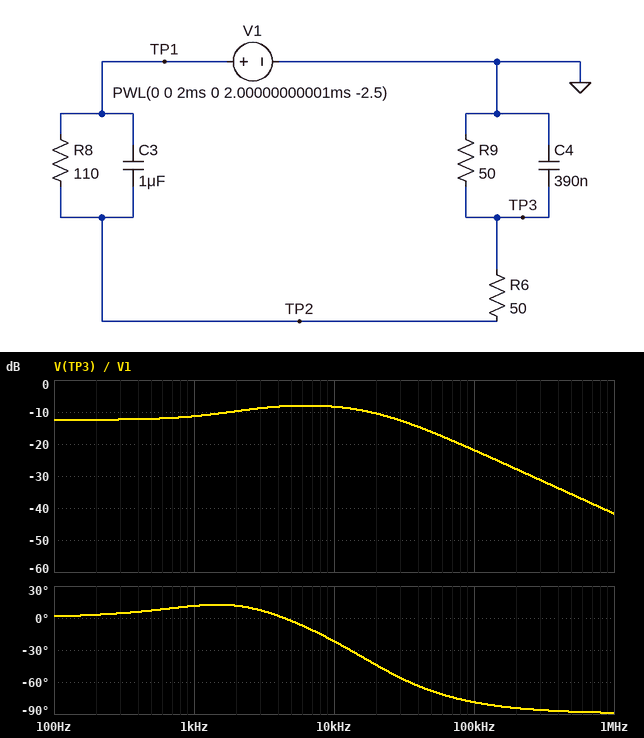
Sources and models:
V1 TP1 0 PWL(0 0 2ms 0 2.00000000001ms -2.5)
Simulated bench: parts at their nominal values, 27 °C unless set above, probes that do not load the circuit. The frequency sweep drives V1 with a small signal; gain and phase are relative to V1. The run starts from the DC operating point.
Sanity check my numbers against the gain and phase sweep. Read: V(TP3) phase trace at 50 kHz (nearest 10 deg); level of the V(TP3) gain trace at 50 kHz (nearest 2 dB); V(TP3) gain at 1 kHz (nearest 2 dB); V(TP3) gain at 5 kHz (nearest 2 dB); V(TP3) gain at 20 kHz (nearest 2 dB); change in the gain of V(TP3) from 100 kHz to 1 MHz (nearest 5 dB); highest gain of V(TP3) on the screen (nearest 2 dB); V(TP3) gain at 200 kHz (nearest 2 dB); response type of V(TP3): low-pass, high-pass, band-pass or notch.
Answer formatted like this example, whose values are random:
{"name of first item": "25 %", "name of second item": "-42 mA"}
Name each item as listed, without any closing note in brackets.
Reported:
{"V(TP3) phase trace at 50 kHz": "-70 deg", "level of the V(TP3) gain trace at 50 kHz": "-16 dB", "V(TP3) gain at 1 kHz": "-12 dB", "V(TP3) gain at 5 kHz": "-8 dB", "V(TP3) gain at 20 kHz": "-10 dB", "change in the gain of V(TP3) from 100 kHz to 1 MHz": "-20 dB", "highest gain of V(TP3) on the screen": "-8 dB", "V(TP3) gain at 200 kHz": "-28 dB", "response type of V(TP3): low-pass, high-pass, band-pass or notch": "low-pass"}
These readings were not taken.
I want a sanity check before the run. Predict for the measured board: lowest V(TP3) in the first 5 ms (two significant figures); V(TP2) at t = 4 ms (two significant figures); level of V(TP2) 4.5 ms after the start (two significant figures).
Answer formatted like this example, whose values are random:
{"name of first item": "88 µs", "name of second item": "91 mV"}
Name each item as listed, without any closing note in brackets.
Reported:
{"lowest V(TP3) in the first 5 ms": "-930 mV", "V(TP2) at t = 4 ms": "-1.2 V", "level of V(TP2) 4.5 ms after the start": "-1.2 V"}
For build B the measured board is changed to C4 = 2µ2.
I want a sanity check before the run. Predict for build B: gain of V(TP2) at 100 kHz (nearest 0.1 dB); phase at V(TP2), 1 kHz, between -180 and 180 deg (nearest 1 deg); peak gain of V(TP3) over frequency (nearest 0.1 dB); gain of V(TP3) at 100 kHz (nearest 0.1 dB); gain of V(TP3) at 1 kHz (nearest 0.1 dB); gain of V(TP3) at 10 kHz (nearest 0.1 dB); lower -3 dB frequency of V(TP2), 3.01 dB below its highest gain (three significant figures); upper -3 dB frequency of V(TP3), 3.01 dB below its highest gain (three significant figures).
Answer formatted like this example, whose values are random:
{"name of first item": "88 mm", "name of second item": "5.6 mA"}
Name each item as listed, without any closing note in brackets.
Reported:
{"gain of V(TP2) at 100 kHz": "0 dB", "phase at V(TP2), 1 kHz, between -180 and 180 deg": "10 deg", "peak gain of V(TP3) over frequency": "-12.5 dB", "gain of V(TP3) at 100 kHz": "-36.8 dB", "gain of V(TP3) at 1 kHz": "-12.6 dB", "gain of V(TP3) at 10 kHz": "-18.2 dB", "lower -3 dB frequency of V(TP2), 3.01 dB below its highest gain": "4.49 kHz", "upper -3 dB frequency of V(TP3), 3.01 dB below its highest gain": "6.08 kHz"}
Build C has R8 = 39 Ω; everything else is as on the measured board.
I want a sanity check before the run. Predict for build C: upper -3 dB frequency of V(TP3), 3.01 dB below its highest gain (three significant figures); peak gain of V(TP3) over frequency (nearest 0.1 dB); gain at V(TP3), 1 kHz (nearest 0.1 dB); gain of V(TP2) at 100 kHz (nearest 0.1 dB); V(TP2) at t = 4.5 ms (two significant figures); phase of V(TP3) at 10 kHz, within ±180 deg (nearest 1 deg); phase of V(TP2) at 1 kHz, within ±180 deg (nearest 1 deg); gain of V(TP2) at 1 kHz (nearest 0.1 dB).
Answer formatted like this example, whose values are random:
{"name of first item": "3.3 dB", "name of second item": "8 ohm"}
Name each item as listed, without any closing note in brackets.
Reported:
{"upper -3 dB frequency of V(TP3), 3.01 dB below its highest gain": "22.9 kHz", "peak gain of V(TP3) over frequency": "-8.2 dB", "gain at V(TP3), 1 kHz": "-8.8 dB", "gain of V(TP2) at 100 kHz": "0 dB", "V(TP2) at t = 4.5 ms": "-1.8 V", "phase of V(TP3) at 10 kHz, within ±180 deg": "-24 deg", "phase of V(TP2) at 1 kHz, within ±180 deg": "3 deg", "gain of V(TP2) at 1 kHz": "-2.8 dB"}
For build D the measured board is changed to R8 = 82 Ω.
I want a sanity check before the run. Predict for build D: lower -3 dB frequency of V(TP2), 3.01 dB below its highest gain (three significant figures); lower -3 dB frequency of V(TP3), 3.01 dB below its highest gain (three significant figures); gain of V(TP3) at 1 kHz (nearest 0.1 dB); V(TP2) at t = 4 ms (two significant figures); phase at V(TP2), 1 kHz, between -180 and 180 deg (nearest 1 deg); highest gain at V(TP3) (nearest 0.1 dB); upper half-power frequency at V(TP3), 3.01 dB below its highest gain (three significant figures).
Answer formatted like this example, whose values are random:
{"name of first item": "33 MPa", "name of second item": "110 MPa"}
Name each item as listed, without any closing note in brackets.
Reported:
{"lower -3 dB frequency of V(TP2), 3.01 dB below its highest gain": "2.55 kHz", "lower -3 dB frequency of V(TP3), 3.01 dB below its highest gain": "452 Hz", "gain of V(TP3) at 1 kHz": "-10.6 dB", "V(TP2) at t = 4 ms": "-1.4 V", "phase at V(TP2), 1 kHz, between -180 and 180 deg": "10 deg", "highest gain at V(TP3)": "-8.1 dB", "upper half-power frequency at V(TP3), 3.01 dB below its highest gain": "22.6 kHz"}
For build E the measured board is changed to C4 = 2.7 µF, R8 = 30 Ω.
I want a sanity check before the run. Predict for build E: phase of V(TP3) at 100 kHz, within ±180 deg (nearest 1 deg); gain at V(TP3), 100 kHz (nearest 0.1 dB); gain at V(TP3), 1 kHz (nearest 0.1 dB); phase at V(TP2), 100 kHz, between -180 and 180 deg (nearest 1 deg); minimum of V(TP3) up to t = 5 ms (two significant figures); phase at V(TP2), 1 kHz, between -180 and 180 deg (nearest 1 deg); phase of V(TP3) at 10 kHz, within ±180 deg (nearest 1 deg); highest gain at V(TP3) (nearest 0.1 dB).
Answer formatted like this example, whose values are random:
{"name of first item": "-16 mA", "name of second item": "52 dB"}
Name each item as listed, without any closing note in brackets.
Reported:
{"phase of V(TP3) at 100 kHz, within ±180 deg": "-87 deg", "gain at V(TP3), 100 kHz": "-38.6 dB", "gain at V(TP3), 1 kHz": "-9.4 dB", "phase at V(TP2), 100 kHz, between -180 and 180 deg": "2 deg", "minimum of V(TP3) up to t = 5 ms": "-960 mV", "phase at V(TP2), 1 kHz, between -180 and 180 deg": "-2 deg", "phase of V(TP3) at 10 kHz, within ±180 deg": "-66 deg", "highest gain at V(TP3)": "-8.3 dB"}
